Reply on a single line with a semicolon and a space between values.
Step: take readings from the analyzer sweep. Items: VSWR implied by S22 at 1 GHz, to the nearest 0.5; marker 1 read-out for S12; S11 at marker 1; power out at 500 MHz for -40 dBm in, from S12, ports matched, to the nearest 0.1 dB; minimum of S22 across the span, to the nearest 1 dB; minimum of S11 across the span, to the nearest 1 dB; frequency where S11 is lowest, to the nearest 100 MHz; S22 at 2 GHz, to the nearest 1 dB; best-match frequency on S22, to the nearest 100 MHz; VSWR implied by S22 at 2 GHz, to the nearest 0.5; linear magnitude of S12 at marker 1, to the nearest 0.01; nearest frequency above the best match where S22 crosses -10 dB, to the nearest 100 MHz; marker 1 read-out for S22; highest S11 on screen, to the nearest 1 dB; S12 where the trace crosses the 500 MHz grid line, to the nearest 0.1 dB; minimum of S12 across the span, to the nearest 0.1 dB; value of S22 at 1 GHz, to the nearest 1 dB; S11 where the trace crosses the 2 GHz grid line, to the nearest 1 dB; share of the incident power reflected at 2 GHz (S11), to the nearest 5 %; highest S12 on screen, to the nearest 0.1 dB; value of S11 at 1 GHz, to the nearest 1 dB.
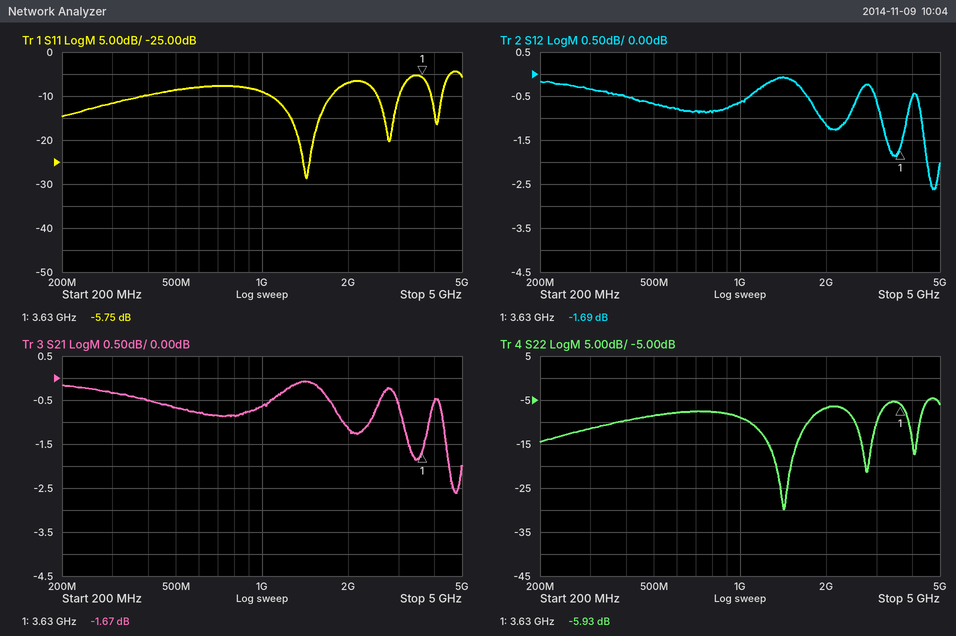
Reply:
2.0; -1.69 dB; -5.75 dB; -40.7 dBm; -30 dB; -29 dB; 1.4 GHz; -7 dB; 1.4 GHz; 2.5; 0.82; 1.7 GHz; -5.93 dB; -4 dB; -0.7 dB; -2.6 dB; -9 dB; -7 dB; 20 %; -0.1 dB; -9 dB
